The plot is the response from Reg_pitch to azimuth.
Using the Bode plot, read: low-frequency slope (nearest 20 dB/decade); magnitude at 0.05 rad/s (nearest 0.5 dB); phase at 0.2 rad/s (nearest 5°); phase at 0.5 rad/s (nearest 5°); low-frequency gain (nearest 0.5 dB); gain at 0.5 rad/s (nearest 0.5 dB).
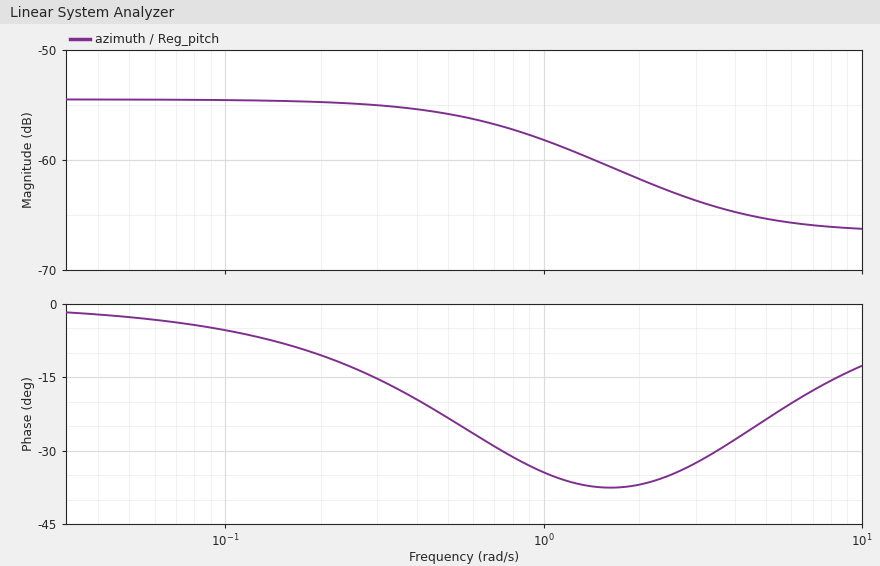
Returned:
0 dB/decade
-54.5 dB
-10°
-25°
-54.5 dB
-56.0 dB
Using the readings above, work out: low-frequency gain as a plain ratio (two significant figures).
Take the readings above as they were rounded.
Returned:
0.0019
